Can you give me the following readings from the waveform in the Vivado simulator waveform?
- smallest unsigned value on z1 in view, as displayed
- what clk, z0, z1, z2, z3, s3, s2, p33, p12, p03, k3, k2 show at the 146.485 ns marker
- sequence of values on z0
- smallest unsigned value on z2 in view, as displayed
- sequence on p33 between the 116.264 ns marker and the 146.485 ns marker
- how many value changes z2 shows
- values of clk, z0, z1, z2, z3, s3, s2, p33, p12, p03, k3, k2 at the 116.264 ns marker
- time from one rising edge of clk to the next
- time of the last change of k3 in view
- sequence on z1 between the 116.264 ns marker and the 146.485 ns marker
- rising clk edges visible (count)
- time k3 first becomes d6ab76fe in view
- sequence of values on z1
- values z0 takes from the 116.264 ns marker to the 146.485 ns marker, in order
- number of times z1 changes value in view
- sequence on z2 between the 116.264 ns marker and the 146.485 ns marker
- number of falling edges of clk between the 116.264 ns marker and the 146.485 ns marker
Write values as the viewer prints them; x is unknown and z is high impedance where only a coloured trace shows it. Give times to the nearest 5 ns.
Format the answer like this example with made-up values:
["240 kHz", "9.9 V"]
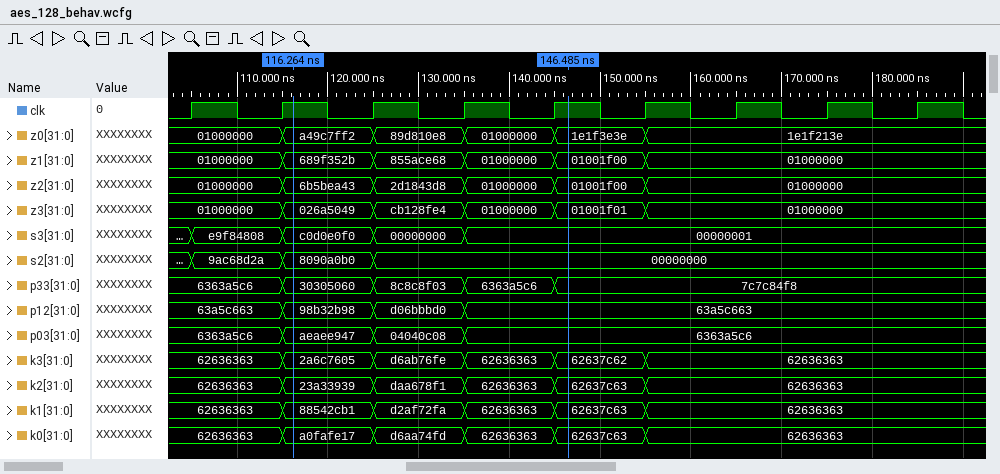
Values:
["01000000", "clk=1, z0=1e1f3e3e, z1=01001f00, z2=01001f00, z3=01001f01, s3=00000001, s2=00000000, p33=7c7c84f8, p12=63a5c663, p03=6363a5c6, k3=62637c62, k2=62637c63", "01000000, a49c7ff2, 89d810e8, 01000000, 1e1f3e3e, 1e1f213e", "01000000", "30305060, 8c8c8f03, 6363a5c6, 7c7c84f8", "5", "clk=1, z0=a49c7ff2, z1=689f352b, z2=6b5bea43, z3=026a5049, s3=c0d0e0f0, s2=8090a0b0, p33=30305060, p12=98b32b98, p03=aeaee947, k3=2a6c7605, k2=23a33939", "10 ns", "155 ns", "689f352b, 855ace68, 01000000, 01001f00", "9", "125 ns", "01000000, 689f352b, 855ace68, 01000000, 01001f00, 01000000", "a49c7ff2, 89d810e8, 01000000, 1e1f3e3e", "5", "6b5bea43, 2d1843d8, 01000000, 01001f00", "3"]
